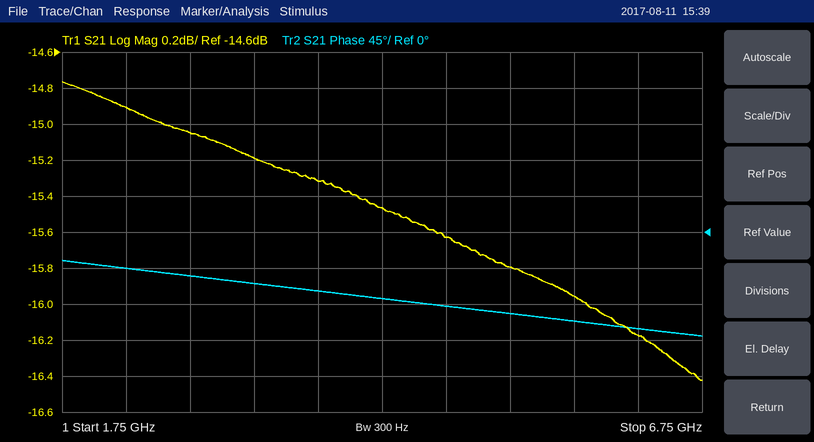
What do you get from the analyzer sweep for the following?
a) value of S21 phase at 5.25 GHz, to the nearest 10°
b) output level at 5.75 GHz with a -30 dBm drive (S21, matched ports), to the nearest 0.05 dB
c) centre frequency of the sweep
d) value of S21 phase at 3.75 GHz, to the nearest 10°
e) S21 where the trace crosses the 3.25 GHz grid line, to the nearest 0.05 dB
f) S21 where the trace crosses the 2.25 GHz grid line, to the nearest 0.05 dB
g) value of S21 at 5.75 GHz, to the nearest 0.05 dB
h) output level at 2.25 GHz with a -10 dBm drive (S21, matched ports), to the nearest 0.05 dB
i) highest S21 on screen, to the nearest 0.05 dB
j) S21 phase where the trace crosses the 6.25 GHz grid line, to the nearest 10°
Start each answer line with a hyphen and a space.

- -100°
- -45.95 dBm
- 4.25 GHz
- -70°
- -15.20 dB
- -14.90 dB
- -15.95 dB
- -24.90 dBm
- -14.75 dB
- -120°
